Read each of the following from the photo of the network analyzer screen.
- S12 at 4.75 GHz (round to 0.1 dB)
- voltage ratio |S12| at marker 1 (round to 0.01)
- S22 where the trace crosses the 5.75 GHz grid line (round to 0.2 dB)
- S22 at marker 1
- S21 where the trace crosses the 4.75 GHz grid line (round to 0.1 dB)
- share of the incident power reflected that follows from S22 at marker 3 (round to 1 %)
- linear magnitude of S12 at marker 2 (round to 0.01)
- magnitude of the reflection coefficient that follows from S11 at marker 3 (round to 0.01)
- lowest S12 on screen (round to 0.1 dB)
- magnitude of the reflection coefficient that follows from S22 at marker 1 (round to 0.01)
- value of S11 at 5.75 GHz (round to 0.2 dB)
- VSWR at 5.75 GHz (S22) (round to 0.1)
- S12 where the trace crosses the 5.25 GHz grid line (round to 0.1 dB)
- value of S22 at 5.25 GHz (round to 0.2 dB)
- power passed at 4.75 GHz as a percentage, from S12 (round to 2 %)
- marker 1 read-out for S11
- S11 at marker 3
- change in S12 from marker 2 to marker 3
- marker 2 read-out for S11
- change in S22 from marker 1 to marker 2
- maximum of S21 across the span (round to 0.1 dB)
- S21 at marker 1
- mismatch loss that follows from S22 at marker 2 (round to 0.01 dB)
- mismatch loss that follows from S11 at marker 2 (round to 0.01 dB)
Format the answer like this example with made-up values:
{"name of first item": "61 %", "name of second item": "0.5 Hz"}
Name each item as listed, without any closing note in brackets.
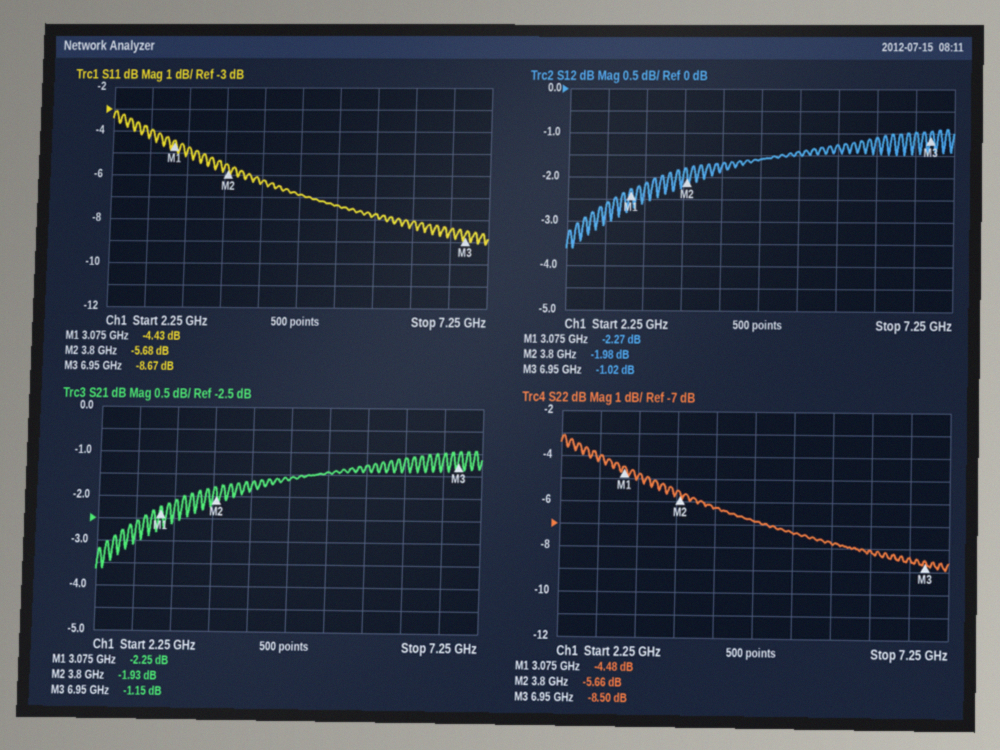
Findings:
{"S12 at 4.75 GHz": "-1.6 dB", "voltage ratio |S12| at marker 1": "0.77", "S22 where the trace crosses the 5.75 GHz grid line": "-7.8 dB", "S22 at marker 1": "-4.48 dB", "S21 where the trace crosses the 4.75 GHz grid line": "-1.6 dB", "share of the incident power reflected that follows from S22 at marker 3": "14 %", "linear magnitude of S12 at marker 2": "0.80", "magnitude of the reflection coefficient that follows from S11 at marker 3": "0.37", "lowest S12 on screen": "-3.6 dB", "magnitude of the reflection coefficient that follows from S22 at marker 1": "0.60", "value of S11 at 5.75 GHz": "-7.8 dB", "VSWR at 5.75 GHz (S22)": "2.4", "S12 where the trace crosses the 5.25 GHz grid line": "-1.4 dB", "value of S22 at 5.25 GHz": "-7.4 dB", "power passed at 4.75 GHz as a percentage, from S12": "70 %", "marker 1 read-out for S11": "-4.43 dB", "S11 at marker 3": "-8.67 dB", "change in S12 from marker 2 to marker 3": "0.96 dB", "marker 2 read-out for S11": "-5.68 dB", "change in S22 from marker 1 to marker 2": "-1.18 dB", "maximum of S21 across the span": "-0.9 dB", "S21 at marker 1": "-2.25 dB", "mismatch loss that follows from S22 at marker 2": "1.38 dB", "mismatch loss that follows from S11 at marker 2": "1.37 dB"}
